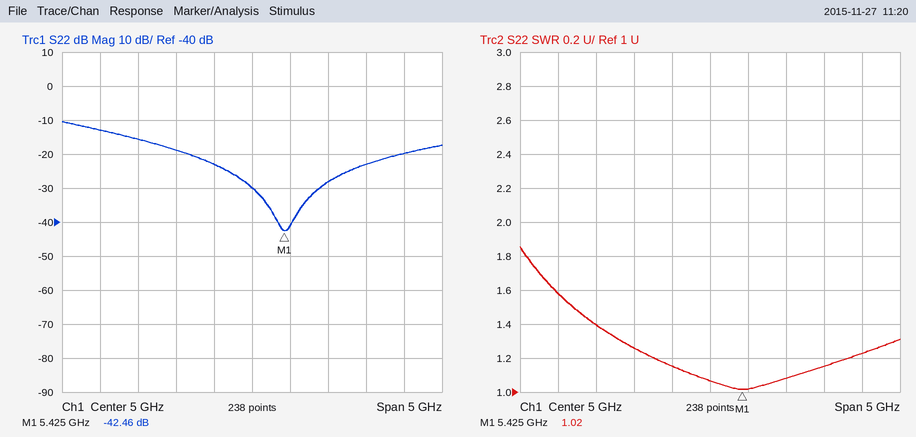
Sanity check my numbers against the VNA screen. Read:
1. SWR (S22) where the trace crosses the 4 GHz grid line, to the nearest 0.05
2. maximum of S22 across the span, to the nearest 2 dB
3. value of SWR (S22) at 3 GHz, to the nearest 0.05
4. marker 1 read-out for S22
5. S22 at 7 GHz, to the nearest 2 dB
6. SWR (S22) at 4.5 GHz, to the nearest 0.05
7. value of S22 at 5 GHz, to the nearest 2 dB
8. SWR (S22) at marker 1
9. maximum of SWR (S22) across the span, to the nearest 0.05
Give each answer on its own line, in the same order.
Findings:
1.25
-10 dB
1.60
-42.46 dB
-20 dB
1.15
-30 dB
1.02
1.85
